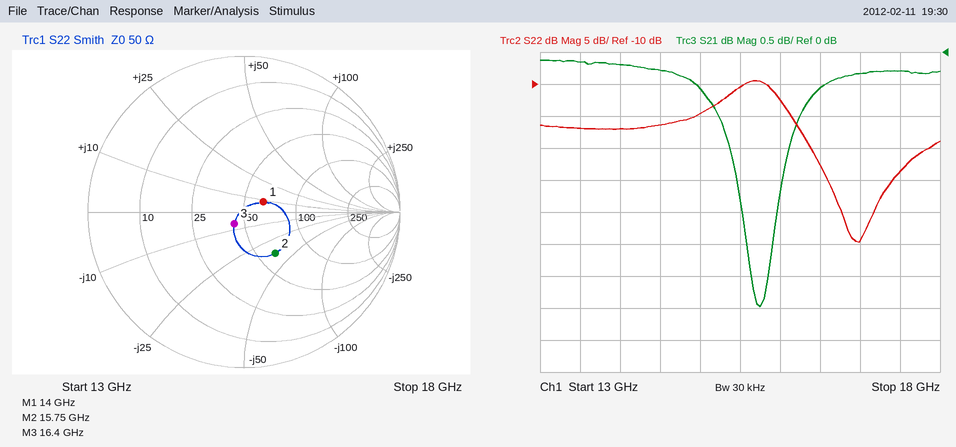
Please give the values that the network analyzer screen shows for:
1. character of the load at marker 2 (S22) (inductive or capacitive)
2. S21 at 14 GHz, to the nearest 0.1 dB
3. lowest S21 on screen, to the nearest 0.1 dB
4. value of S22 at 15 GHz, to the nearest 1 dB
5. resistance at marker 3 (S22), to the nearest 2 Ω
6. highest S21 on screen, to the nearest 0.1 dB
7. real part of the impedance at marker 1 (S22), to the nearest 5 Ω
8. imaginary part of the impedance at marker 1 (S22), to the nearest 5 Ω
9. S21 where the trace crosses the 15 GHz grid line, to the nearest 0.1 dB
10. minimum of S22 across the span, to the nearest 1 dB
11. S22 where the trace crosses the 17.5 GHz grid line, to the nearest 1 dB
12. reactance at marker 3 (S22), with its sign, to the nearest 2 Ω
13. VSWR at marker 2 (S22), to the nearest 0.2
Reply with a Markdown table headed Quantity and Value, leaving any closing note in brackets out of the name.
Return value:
| Quantity | Value |
|---|---|
| character of the load at marker 2 (S22) | capacitive |
| S21 at 14 GHz, to the nearest 0.1 dB | -0.2 dB |
| lowest S21 on screen, to the nearest 0.1 dB | -4.0 dB |
| value of S22 at 15 GHz, to the nearest 1 dB | -15 dB |
| resistance at marker 3 (S22), to the nearest 2 Ω | 44 Ω |
| highest S21 on screen, to the nearest 0.1 dB | -0.1 dB |
| real part of the impedance at marker 1 (S22), to the nearest 5 Ω | 65 Ω |
| imaginary part of the impedance at marker 1 (S22), to the nearest 5 Ω | +10 Ω |
| S21 where the trace crosses the 15 GHz grid line, to the nearest 0.1 dB | -0.6 dB |
| minimum of S22 across the span, to the nearest 1 dB | -35 dB |
| S22 where the trace crosses the 17.5 GHz grid line, to the nearest 1 dB | -24 dB |
| reactance at marker 3 (S22), with its sign, to the nearest 2 Ω | -6 Ω |
| VSWR at marker 2 (S22), to the nearest 0.2 | 2.0 |
